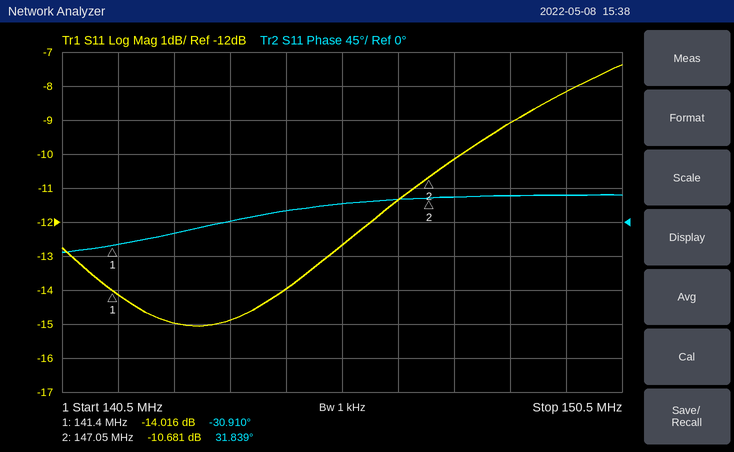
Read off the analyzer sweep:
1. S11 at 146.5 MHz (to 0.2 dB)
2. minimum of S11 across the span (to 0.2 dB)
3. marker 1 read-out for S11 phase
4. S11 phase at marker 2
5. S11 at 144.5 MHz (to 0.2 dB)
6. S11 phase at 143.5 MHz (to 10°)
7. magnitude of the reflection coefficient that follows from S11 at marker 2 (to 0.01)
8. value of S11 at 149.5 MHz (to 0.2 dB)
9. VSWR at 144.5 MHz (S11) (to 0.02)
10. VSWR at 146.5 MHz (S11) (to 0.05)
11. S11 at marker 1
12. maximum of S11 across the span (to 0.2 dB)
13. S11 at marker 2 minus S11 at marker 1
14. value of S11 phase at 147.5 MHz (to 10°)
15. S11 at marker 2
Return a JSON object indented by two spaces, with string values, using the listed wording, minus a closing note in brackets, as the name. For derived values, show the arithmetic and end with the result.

{
  "S11 at 146.5 MHz": "-11.4 dB",
  "minimum of S11 across the span": "-15.0 dB",
  "marker 1 read-out for S11 phase": "-30.910°",
  "S11 phase at marker 2": "31.839°",
  "S11 at 144.5 MHz": "-14.0 dB",
  "S11 phase at 143.5 MHz": "0°",
  "magnitude of the reflection coefficient that follows from S11 at marker 2": "10^(-10.681/20) ≈ 0.29",
  "value of S11 at 149.5 MHz": "-8.2 dB",
  "VSWR at 144.5 MHz (S11)": "|Γ| = 10^(-14/20) = 0.1995; VSWR = (1 + 0.1995)/(1 − 0.1995) ≈ 1.50",
  "VSWR at 146.5 MHz (S11)": "|Γ| = 10^(-11.4/20) = 0.2692; VSWR = (1 + 0.2692)/(1 − 0.2692) ≈ 1.74, so 1.75 to the nearest 0.05",
  "S11 at marker 1": "-14.016 dB",
  "maximum of S11 across the span": "-7.4 dB",
  "S11 at marker 2 minus S11 at marker 1": "-10.681 − (-14.016) = 3.335 dB",
  "value of S11 phase at 147.5 MHz": "30°",
  "S11 at marker 2": "-10.681 dB"
}
